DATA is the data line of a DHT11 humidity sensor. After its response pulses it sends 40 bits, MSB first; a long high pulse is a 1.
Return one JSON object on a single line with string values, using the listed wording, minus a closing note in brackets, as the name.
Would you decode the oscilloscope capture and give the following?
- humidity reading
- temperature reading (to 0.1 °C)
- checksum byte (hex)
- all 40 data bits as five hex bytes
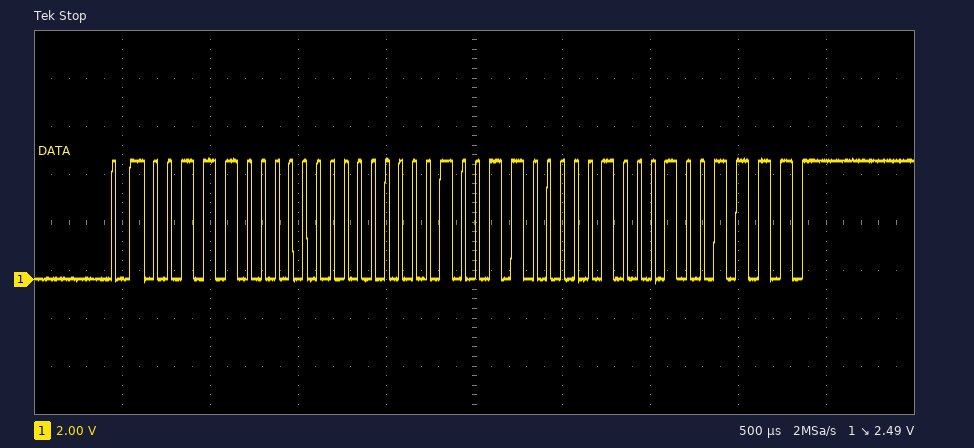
{"humidity reading": "56 %", "temperature reading": "19.4 °C", "checksum byte": "0x4F", "all 40 data bits as five hex bytes": "38 00 13 04 4F"}
